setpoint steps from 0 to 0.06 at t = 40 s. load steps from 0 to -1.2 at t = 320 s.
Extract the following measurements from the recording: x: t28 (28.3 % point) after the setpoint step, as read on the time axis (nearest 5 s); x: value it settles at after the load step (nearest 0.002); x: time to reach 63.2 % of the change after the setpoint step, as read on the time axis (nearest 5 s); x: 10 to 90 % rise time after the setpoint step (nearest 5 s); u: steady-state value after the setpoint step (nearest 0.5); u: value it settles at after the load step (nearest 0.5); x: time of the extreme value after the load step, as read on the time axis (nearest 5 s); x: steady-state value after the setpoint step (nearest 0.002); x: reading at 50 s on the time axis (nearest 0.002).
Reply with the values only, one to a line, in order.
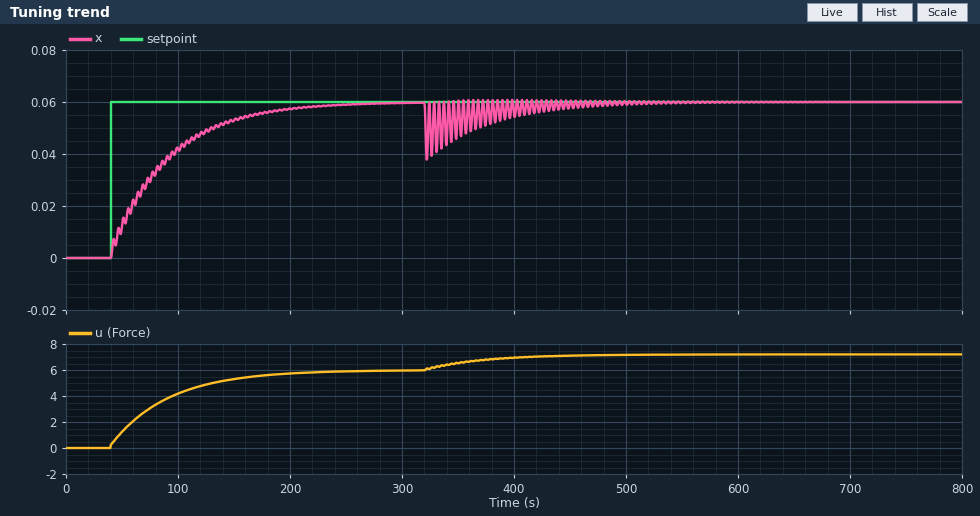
55 s
0.060
90 s
115 s
6.0
7.0
320 s
0.060
0.012
